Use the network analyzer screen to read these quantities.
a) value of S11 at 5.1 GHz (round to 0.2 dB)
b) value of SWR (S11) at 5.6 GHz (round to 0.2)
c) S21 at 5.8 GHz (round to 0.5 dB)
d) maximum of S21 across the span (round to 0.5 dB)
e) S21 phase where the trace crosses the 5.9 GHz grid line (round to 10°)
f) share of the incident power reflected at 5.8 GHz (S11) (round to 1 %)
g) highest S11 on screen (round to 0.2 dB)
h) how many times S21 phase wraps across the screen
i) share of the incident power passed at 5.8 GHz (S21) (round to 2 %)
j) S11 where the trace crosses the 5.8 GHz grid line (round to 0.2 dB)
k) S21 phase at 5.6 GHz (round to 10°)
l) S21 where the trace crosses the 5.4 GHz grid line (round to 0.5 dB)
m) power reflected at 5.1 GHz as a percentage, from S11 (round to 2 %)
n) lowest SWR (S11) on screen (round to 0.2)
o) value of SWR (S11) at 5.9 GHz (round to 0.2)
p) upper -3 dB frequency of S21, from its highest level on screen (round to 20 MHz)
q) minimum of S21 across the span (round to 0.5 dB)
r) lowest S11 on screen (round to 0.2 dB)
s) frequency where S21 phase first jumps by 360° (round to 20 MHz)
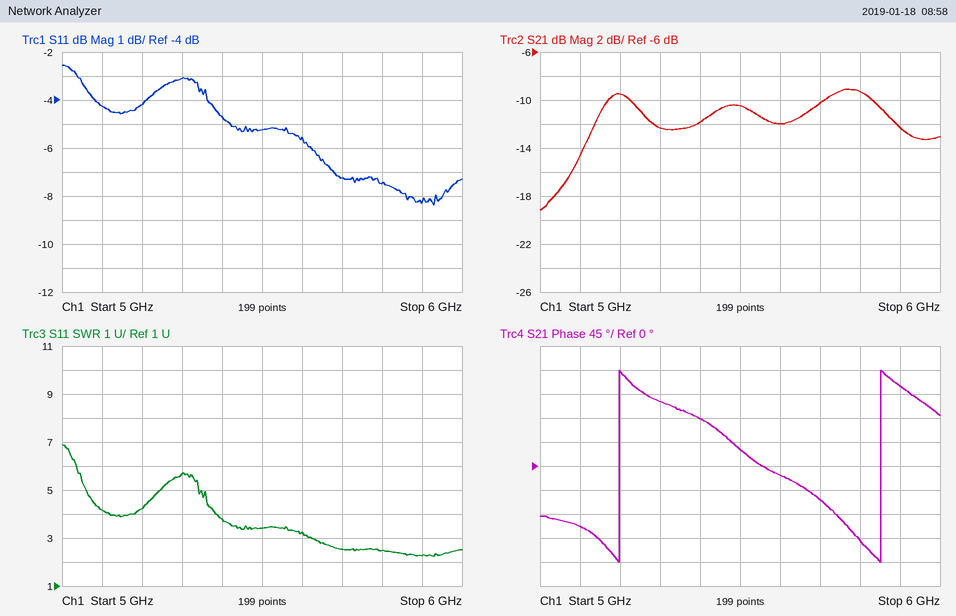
-4.2 dB
3.2
-9.5 dB
-9.0 dB
150°
18 %
-2.6 dB
2
12 %
-7.4 dB
-20°
-12.0 dB
38 %
2.2
2.2
5.90 GHz
-19.0 dB
-8.4 dB
5.20 GHz
